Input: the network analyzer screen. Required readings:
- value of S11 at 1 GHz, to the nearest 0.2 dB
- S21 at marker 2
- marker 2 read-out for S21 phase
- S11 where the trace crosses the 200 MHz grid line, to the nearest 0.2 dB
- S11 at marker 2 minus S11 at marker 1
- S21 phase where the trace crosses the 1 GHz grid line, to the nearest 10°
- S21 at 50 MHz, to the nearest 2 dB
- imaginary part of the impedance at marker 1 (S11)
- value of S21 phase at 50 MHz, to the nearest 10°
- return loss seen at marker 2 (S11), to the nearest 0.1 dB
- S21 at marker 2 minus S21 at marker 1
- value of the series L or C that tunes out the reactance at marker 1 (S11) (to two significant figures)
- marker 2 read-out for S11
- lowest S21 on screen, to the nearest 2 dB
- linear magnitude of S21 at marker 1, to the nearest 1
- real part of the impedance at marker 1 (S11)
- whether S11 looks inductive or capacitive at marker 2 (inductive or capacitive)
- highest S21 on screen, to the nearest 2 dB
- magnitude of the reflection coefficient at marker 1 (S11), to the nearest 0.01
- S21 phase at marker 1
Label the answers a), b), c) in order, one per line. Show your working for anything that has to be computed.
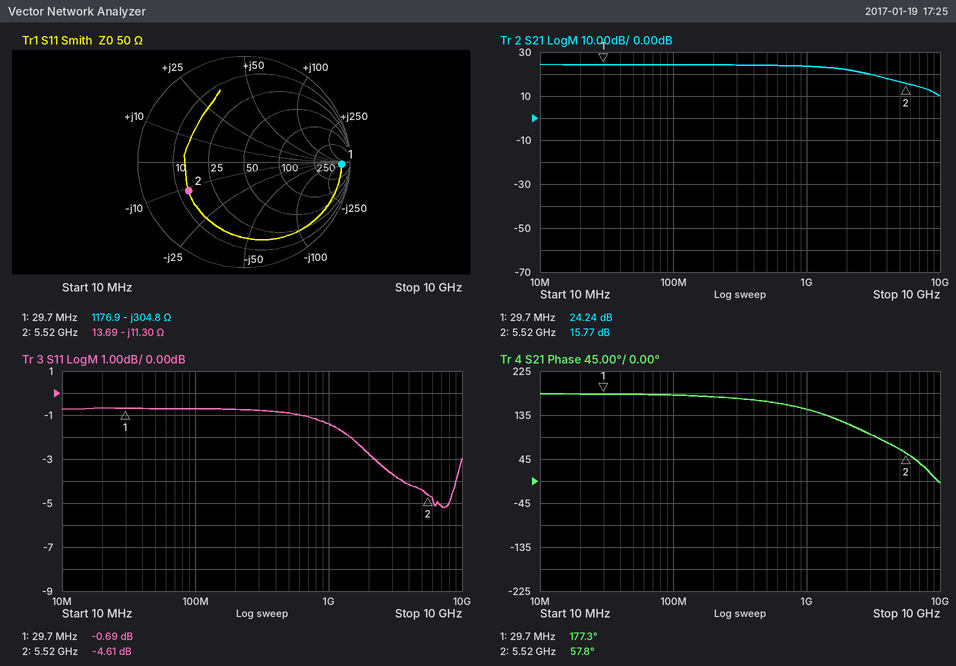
a) -1.4 dB
b) 15.77 dB
c) 57.8°
d) -0.8 dB
e) -4.61 − (-0.69) = -3.92 dB
f) 150°
g) 24 dB
h) -304.8 Ω
i) 180°
j) 4.6 dB
k) 15.77 − (24.24) = -8.47 dB
l) L = 304.8 Ω/(2π × 29.7 MHz) ≈ 1.6 µH
m) -4.61 dB
n) 10 dB
o) 10^(24.24/20) ≈ 16
p) 1176.9 Ω
q) capacitive
r) 24 dB
s) 0.92
t) 177.3°
